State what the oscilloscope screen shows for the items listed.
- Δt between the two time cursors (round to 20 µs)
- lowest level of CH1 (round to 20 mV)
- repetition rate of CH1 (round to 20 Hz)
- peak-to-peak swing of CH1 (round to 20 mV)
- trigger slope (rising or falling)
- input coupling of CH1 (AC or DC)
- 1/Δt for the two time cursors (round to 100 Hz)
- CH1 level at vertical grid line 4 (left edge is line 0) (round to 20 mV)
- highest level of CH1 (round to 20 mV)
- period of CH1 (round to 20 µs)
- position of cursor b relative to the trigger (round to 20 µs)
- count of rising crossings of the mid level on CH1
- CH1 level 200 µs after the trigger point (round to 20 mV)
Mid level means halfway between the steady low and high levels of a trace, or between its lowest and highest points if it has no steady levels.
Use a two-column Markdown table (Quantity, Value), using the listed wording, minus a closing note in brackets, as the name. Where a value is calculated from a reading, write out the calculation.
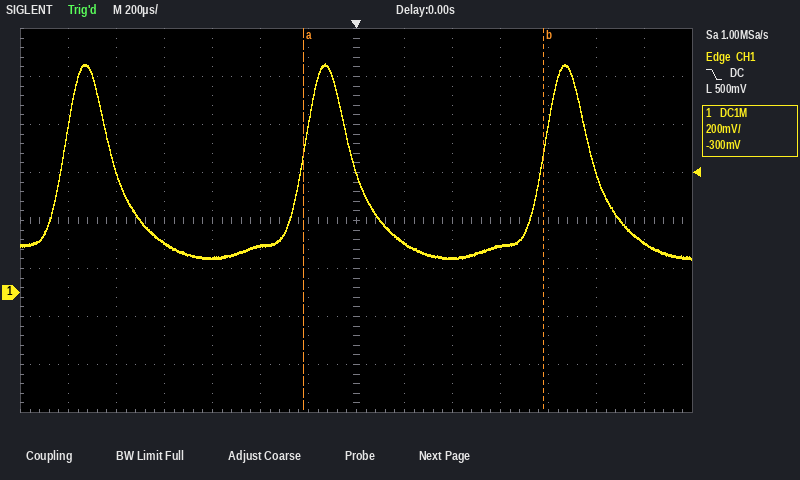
| Quantity | Value |
|---|---|
| Δt between the two time cursors | 1.00 ms |
| lowest level of CH1 | 140 mV |
| repetition rate of CH1 | 1 / 1.00 ms ≈ 1.00 kHz |
| peak-to-peak swing of CH1 | 960 mV − (140 mV) = 820 mV |
| trigger slope | falling |
| input coupling of CH1 | DC |
| 1/Δt for the two time cursors | 1 / 1.00 ms ≈ 1.0 kHz |
| CH1 level at vertical grid line 4 (left edge is line 0) | 140 mV |
| highest level of CH1 | 960 mV |
| period of CH1 | 1.00 ms |
| position of cursor b relative to the trigger | +780 µs |
| count of rising crossings of the mid level on CH1 | 3 |
| CH1 level 200 µs after the trigger point | 200 mV |
